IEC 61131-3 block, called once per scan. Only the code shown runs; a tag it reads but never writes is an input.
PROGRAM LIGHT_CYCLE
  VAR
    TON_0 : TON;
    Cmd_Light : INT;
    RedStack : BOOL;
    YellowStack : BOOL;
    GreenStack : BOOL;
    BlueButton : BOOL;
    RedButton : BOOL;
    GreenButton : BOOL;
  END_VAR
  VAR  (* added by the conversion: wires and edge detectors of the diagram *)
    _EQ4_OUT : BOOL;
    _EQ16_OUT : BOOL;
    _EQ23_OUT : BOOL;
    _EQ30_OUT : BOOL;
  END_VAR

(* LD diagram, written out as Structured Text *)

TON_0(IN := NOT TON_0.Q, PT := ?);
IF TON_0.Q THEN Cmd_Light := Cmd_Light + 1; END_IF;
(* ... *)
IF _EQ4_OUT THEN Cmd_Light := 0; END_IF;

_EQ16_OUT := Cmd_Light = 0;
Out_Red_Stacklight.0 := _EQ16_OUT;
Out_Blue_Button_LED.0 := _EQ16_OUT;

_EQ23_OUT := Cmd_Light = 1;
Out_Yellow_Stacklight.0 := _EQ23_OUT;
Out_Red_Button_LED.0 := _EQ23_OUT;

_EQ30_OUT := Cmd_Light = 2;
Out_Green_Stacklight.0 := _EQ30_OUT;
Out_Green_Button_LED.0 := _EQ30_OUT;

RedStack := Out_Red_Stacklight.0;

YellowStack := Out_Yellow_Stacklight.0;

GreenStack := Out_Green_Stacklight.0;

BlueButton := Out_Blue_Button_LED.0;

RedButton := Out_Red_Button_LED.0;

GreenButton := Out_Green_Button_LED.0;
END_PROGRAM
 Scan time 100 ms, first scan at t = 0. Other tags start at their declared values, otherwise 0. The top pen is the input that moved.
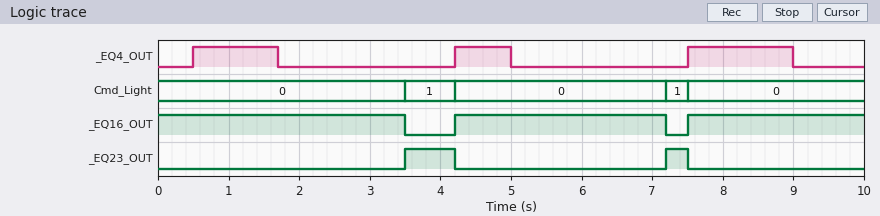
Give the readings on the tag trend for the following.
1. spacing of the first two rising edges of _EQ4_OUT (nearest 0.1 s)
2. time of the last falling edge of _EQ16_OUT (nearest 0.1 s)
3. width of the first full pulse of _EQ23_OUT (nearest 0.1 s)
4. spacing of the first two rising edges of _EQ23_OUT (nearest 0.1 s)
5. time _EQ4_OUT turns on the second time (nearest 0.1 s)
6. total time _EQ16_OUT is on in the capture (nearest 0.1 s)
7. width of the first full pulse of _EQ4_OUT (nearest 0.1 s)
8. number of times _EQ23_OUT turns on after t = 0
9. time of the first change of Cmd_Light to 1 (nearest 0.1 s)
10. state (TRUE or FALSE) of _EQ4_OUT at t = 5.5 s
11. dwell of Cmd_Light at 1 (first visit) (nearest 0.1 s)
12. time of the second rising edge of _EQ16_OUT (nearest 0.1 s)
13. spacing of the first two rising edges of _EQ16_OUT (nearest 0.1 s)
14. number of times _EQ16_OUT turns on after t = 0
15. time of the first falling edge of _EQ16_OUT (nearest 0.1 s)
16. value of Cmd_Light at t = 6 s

3.7 s
7.2 s
0.7 s
3.7 s
4.2 s
9.0 s
1.2 s
2
3.5 s
FALSE
0.7 s
7.5 s
3.3 s
2
3.5 s
0
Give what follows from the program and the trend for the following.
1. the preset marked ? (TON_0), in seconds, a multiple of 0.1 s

3.5 s
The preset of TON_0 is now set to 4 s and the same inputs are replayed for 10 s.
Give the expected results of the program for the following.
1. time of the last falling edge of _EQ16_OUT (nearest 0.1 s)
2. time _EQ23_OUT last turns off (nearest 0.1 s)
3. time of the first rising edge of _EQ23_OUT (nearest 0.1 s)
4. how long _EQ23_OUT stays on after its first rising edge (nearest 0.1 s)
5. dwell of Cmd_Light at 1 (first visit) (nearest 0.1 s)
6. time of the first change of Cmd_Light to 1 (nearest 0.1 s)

4.0 s
4.2 s
4.0 s
0.2 s
0.2 s
4.0 s
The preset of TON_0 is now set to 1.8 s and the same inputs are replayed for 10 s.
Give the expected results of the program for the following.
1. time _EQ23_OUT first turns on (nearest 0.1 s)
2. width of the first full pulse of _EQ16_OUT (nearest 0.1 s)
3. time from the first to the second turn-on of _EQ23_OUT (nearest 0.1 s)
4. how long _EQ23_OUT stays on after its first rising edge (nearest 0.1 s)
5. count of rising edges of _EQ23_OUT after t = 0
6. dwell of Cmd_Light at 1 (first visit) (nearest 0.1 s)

1.8 s
1.6 s
4.0 s
2.0 s
3
2.0 s
